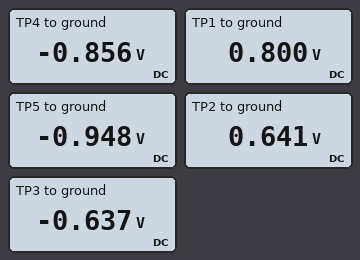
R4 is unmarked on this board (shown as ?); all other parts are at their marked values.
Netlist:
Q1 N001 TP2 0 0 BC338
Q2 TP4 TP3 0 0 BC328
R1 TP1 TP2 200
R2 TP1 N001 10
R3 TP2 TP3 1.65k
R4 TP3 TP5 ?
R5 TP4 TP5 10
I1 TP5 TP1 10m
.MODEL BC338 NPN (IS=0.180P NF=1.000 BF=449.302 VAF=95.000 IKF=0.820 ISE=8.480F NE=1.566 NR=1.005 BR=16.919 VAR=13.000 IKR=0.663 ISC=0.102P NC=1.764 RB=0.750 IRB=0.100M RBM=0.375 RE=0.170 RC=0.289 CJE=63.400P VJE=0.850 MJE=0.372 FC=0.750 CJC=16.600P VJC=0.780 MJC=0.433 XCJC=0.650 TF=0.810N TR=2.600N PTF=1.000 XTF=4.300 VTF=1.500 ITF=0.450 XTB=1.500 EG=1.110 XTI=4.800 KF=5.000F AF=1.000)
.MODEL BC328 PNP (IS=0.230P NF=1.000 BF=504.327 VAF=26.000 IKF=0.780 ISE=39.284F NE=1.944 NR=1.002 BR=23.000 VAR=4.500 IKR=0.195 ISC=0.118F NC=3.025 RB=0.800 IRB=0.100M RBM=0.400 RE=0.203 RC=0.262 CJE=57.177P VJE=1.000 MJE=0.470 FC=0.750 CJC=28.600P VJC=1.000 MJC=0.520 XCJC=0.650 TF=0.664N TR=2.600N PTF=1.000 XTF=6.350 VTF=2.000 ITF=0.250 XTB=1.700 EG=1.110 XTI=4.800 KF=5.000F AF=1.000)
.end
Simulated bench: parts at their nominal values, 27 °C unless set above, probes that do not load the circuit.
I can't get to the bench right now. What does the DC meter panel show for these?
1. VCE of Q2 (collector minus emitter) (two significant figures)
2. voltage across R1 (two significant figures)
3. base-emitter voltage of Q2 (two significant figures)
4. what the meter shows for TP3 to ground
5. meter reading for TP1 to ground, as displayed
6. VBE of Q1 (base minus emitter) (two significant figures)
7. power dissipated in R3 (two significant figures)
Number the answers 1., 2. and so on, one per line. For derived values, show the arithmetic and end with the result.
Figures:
1. -856 mV = -860 mV
2. 800 mV - 641 mV = 160 mV
3. -637 mV = -640 mV
4. -0.637 V
5. 0.800 V
6. 641 mV = 640 mV
7. (641 mV - (-637 mV))^2 / 1.65 kΩ = 990 µW
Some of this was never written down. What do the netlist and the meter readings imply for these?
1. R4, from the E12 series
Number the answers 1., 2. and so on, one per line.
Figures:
1. 390 Ω
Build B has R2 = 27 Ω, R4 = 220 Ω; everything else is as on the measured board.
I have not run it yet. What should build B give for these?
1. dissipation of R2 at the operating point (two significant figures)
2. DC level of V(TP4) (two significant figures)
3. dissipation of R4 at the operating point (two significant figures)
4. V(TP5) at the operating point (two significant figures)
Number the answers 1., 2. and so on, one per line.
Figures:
1. 2.3 mW
2. -720 mV
3. 140 µW
4. -810 mV
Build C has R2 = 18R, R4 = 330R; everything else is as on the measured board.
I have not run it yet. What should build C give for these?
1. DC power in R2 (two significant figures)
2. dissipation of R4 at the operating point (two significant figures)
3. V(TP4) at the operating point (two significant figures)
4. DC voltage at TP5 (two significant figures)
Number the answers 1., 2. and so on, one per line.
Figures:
1. 1.5 mW
2. 210 µW
3. -810 mV
4. -900 mV
